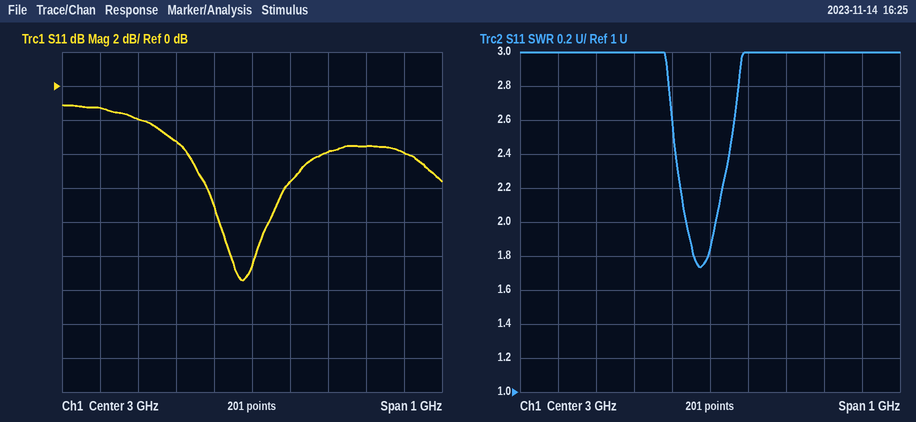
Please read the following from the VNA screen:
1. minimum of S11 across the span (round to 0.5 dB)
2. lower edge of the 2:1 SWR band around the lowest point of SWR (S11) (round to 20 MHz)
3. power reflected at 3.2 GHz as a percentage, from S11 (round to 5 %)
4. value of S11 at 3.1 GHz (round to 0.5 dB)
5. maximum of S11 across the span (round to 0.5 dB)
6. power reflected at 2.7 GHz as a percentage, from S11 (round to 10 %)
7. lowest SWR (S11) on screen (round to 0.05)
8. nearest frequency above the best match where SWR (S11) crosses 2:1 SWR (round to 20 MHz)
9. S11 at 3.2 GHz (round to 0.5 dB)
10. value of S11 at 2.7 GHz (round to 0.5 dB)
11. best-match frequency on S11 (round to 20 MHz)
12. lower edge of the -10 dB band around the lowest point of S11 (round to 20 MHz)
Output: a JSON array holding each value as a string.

["-11.5 dB", "2.94 GHz", "40 %", "-5.5 dB", "-1.0 dB", "60 %", "1.75", "3.02 GHz", "-4.0 dB", "-2.0 dB", "2.98 GHz", "2.94 GHz"]
